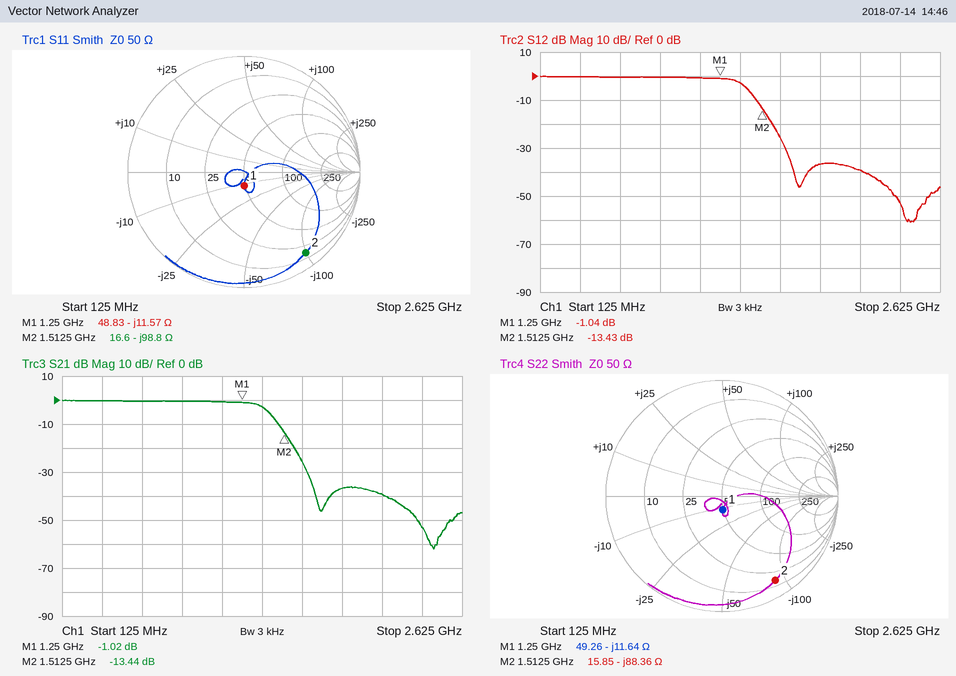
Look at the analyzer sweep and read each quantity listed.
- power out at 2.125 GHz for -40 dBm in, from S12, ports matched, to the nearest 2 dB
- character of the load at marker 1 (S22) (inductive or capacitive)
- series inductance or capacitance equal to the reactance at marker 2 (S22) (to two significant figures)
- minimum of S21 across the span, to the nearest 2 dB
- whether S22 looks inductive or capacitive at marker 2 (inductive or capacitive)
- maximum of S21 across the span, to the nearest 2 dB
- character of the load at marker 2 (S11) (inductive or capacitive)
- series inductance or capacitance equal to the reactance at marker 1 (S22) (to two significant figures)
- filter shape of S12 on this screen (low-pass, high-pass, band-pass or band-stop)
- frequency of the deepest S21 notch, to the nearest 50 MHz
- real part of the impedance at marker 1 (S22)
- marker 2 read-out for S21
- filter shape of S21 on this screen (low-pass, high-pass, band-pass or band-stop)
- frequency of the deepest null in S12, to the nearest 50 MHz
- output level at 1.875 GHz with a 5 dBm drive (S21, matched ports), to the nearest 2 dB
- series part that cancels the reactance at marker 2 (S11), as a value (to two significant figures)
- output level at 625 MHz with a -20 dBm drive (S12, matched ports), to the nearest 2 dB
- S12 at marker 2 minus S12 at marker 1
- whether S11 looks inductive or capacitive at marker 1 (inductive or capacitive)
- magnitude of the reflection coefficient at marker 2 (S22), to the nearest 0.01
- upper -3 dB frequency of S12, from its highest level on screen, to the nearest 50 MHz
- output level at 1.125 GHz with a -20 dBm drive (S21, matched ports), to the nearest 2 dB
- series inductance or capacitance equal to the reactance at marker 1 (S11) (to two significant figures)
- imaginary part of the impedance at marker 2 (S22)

-80 dBm
capacitive
1.2 pF
-62 dB
capacitive
0 dB
capacitive
11 pF
low-pass
2.45 GHz
49.26 Ω
-13.44 dB
low-pass
2.45 GHz
-32 dBm
10 nH
-20 dBm
-12.39 dB
capacitive
0.86
1.40 GHz
-20 dBm
11 pF
-88.36 Ω
